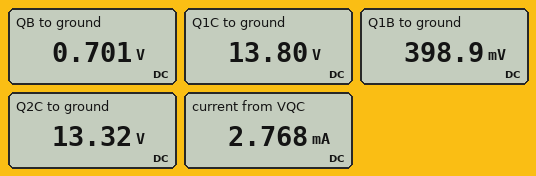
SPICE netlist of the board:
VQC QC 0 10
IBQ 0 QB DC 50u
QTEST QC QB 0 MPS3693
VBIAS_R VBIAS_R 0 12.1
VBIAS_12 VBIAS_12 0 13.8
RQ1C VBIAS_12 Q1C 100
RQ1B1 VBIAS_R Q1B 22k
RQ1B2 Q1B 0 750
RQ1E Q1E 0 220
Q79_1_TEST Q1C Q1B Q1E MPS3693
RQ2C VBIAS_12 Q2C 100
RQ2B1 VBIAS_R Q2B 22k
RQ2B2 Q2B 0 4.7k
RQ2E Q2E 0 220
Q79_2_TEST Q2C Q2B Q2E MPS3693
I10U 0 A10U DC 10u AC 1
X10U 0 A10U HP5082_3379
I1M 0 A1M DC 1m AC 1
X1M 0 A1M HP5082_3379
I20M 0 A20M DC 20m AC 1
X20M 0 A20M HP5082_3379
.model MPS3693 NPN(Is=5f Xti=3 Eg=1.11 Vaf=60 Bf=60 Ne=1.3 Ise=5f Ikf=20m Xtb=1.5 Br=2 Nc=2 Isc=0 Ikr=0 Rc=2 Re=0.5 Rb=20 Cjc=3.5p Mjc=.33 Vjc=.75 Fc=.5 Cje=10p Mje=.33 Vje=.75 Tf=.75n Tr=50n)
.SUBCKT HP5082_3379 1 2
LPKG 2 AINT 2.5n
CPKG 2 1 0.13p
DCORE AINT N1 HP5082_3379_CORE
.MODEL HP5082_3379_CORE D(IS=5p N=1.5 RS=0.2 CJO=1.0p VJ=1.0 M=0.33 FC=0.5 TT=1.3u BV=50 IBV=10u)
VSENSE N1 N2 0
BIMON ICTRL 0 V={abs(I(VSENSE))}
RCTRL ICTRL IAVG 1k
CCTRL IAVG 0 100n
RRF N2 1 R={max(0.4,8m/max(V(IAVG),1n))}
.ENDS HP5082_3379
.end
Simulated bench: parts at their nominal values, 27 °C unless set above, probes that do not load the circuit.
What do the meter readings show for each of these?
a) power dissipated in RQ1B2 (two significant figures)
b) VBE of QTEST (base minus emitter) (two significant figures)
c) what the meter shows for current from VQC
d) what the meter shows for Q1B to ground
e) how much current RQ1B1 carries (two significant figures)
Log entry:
210 µW
700 mV
2.768 mA
398.9 mV
530 µA
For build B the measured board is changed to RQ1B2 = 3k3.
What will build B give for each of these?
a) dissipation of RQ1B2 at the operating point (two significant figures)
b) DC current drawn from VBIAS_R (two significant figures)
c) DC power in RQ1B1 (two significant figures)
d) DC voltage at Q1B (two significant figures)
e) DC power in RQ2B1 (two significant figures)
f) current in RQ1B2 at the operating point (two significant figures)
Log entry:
610 µW
950 µA
5.2 mW
1.4 V
4.8 mW
430 µA
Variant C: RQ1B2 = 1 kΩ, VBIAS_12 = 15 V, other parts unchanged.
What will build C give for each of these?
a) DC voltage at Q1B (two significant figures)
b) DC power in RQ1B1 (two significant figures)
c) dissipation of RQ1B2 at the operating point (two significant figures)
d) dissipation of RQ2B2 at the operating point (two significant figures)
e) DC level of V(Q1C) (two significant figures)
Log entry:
530 mV
6.1 mW
280 µW
680 µW
15 V
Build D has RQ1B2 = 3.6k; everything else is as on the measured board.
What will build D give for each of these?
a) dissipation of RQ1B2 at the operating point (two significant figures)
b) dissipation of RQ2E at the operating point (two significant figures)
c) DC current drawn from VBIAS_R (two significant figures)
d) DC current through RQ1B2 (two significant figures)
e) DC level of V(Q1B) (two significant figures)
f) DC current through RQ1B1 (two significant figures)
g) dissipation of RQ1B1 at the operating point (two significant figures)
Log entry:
630 µW
5.2 mW
950 µA
420 µA
1.5 V
480 µA
5.1 mW
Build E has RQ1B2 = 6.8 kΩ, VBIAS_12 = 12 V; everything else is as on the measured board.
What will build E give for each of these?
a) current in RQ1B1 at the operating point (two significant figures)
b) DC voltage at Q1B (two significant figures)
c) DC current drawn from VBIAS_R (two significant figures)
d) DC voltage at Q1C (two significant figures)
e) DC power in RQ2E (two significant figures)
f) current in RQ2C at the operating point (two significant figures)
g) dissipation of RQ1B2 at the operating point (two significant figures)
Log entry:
450 µA
2.2 V
920 µA
11 V
5.1 mW
4.7 mA
700 µW
